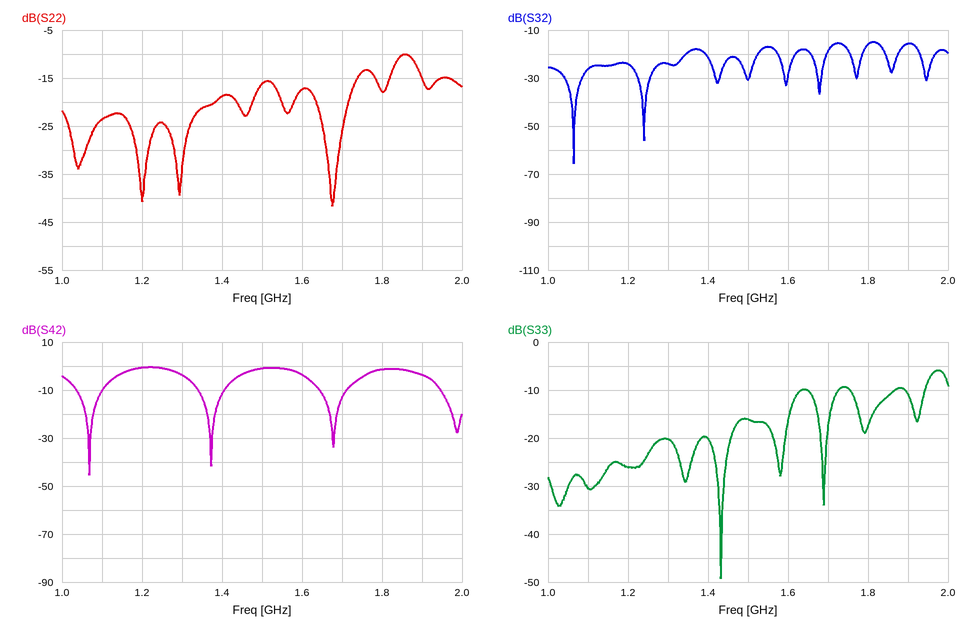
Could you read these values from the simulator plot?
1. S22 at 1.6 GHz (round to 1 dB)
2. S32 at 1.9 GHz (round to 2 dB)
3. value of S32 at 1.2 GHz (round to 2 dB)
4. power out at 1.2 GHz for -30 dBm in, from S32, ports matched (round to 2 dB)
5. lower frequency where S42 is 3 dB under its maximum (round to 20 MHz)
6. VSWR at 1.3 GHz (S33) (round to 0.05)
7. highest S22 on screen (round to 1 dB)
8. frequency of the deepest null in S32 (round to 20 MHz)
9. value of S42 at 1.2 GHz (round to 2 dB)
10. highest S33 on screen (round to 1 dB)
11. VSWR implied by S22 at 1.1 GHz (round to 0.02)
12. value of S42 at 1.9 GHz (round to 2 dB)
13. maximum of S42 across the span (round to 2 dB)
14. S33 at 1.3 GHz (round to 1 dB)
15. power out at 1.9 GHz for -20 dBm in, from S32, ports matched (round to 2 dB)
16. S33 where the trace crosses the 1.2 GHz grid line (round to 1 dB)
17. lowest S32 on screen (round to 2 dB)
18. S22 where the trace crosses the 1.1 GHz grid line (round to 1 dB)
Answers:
-17 dB
-16 dB
-24 dB
-54 dBm
1.14 GHz
1.20
-10 dB
1.06 GHz
0 dB
-6 dB
1.14
-4 dB
0 dB
-20 dB
-36 dBm
-26 dB
-66 dB
-24 dB
